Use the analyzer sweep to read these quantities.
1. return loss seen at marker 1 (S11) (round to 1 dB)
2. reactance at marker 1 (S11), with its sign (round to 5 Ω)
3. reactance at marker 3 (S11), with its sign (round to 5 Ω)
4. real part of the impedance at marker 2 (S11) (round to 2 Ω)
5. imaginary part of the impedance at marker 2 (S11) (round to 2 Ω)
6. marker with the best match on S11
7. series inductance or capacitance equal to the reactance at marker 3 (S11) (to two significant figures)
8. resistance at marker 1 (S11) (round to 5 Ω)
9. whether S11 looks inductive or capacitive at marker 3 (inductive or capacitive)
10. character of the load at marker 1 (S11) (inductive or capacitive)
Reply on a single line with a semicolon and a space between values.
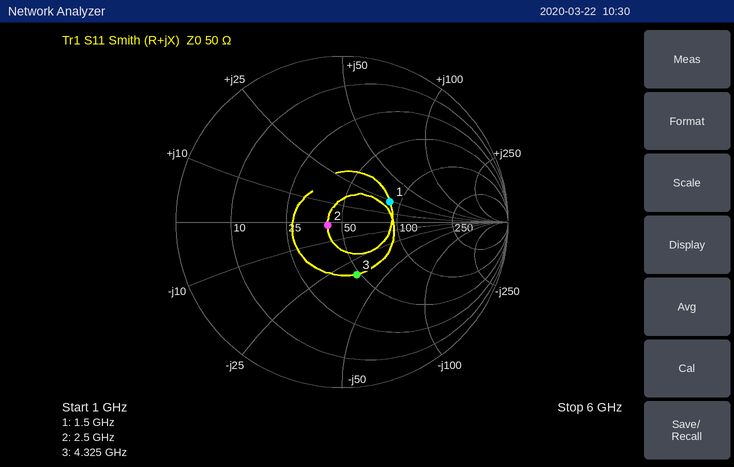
10 dB; +25 Ω; -35 Ω; 42 Ω; -2 Ω; marker 2; 1.1 pF; 85 Ω; capacitive; inductive
